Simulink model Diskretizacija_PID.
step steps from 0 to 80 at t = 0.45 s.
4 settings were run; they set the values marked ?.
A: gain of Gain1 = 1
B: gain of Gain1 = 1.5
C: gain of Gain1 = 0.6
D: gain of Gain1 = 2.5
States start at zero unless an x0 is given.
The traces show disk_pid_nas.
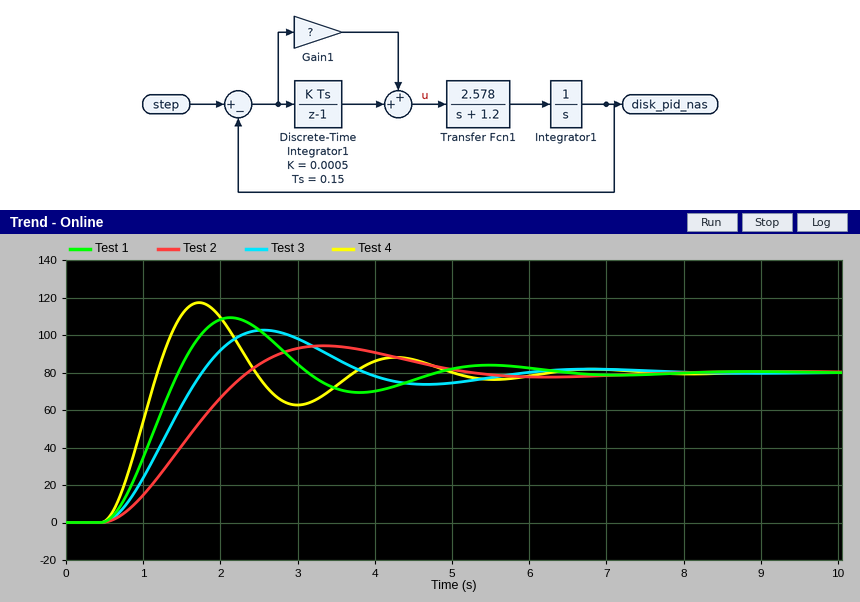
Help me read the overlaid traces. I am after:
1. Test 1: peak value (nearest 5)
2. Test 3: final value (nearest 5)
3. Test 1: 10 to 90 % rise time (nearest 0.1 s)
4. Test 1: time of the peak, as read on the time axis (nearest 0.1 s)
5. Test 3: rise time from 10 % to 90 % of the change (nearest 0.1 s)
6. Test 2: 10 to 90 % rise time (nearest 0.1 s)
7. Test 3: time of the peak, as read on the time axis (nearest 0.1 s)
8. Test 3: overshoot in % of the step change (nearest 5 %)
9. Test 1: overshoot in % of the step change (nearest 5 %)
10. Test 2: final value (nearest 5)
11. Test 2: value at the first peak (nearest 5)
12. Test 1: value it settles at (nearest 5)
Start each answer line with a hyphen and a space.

- 110
- 80
- 0.7 s
- 2.1 s
- 0.9 s
- 1.3 s
- 2.6 s
- 30 %
- 35 %
- 80
- 95
- 80
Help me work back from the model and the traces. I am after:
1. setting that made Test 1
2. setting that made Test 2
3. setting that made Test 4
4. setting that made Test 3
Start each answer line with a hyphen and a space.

- B
- C
- D
- A
